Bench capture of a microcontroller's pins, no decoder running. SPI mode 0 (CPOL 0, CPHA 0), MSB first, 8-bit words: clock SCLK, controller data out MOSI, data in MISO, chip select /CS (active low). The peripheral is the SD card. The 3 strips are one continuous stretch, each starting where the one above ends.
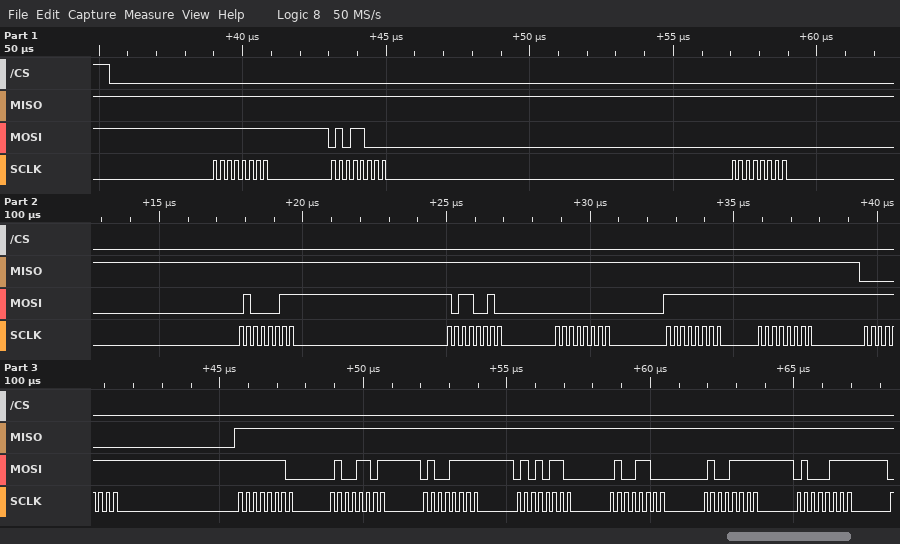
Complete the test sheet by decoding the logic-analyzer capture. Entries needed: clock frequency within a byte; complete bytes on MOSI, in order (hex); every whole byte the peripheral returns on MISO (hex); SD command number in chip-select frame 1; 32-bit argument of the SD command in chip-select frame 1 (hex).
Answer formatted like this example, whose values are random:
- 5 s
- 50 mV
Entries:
- 4 MHz
- FF 58 00 43 B2 00 FF FF FF FE 4D 4F 56 4C 4F 47
- FF FF FF FF FF FF FF FF 00 FF FF FF FF FF FF FF
- CMD24
- 0x0043B200
